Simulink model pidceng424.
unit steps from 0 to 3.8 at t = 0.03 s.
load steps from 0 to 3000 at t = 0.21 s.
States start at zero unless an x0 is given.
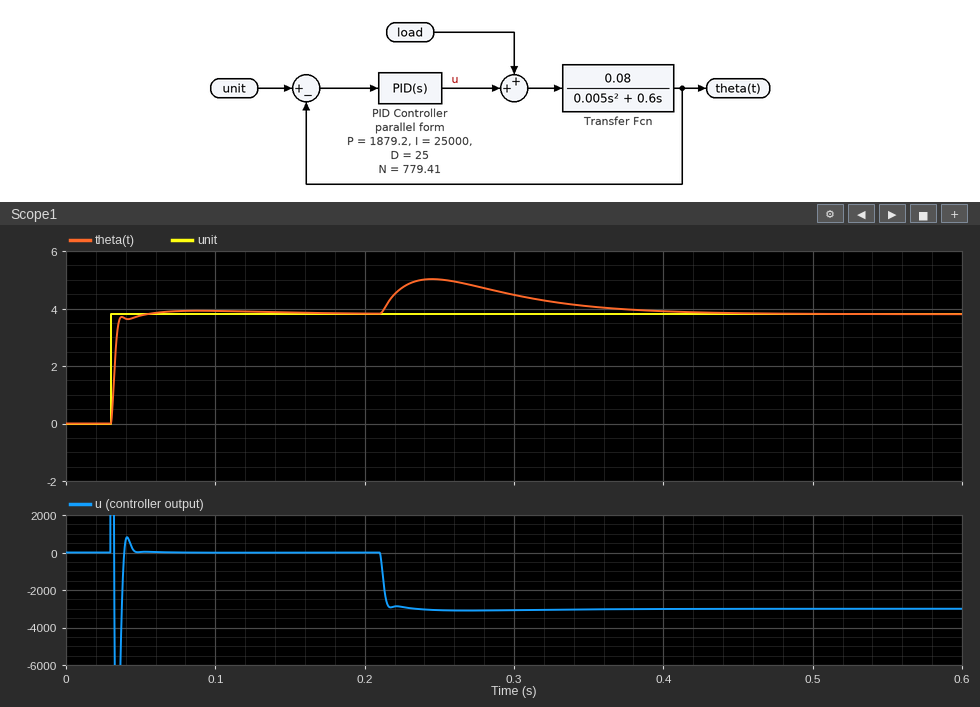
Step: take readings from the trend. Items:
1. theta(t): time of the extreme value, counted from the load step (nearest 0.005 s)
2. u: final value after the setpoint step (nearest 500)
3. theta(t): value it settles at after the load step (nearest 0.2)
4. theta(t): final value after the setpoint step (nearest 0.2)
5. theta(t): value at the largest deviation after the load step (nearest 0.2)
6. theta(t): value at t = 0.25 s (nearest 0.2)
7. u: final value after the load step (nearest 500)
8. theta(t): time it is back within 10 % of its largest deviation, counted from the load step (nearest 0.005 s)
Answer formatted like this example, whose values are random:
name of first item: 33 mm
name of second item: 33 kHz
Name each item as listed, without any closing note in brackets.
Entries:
theta(t): time of the extreme value, counted from the load step: 0.035 s
u: final value after the setpoint step: 0
theta(t): value it settles at after the load step: 3.8
theta(t): final value after the setpoint step: 3.8
theta(t): value at the largest deviation after the load step: 5.0
theta(t): value at t = 0.25 s: 5.0
u: final value after the load step: -3000
theta(t): time it is back within 10 % of its largest deviation, counted from the load step: 0.185 s
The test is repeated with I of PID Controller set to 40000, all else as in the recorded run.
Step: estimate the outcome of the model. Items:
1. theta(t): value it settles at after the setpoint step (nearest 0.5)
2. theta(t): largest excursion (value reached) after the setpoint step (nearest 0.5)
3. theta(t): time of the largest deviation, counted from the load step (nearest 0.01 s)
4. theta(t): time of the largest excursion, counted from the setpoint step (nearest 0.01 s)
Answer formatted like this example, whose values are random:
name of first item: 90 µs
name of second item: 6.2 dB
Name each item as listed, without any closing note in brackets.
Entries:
theta(t): value it settles at after the setpoint step: 4.0
theta(t): largest excursion (value reached) after the setpoint step: 4.0
theta(t): time of the largest deviation, counted from the load step: 0.03 s
theta(t): time of the largest excursion, counted from the setpoint step: 0.05 s
